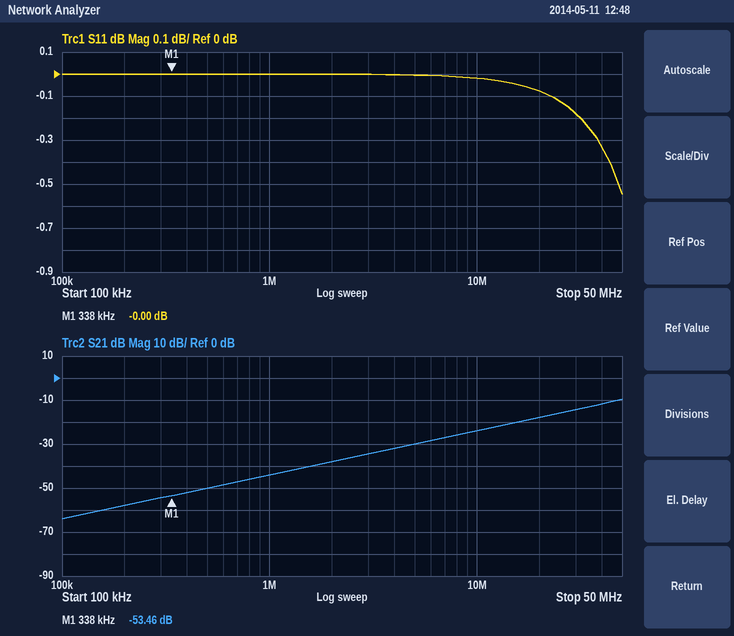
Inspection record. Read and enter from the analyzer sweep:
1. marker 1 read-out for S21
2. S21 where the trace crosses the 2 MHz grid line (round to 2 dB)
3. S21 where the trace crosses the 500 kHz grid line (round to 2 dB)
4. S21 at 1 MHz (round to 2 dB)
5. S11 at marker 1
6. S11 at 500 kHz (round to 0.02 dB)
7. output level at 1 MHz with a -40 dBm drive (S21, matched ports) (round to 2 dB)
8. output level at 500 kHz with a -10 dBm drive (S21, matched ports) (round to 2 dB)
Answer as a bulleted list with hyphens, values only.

- -53.46 dB
- -38 dB
- -50 dB
- -44 dB
- -0.00 dB
- 0.00 dB
- -84 dBm
- -60 dBm
